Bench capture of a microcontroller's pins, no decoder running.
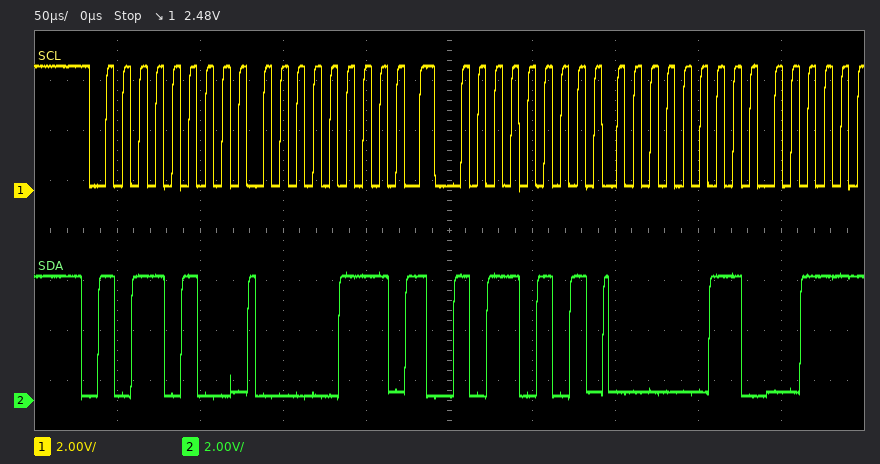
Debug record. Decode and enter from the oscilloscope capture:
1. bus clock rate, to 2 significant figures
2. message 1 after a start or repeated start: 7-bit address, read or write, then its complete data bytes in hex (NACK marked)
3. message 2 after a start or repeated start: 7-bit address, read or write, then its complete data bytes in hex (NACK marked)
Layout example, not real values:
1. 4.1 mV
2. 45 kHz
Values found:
1. 100 kHz
2. 0x5A write: 07
3. 0x5A read: 03
